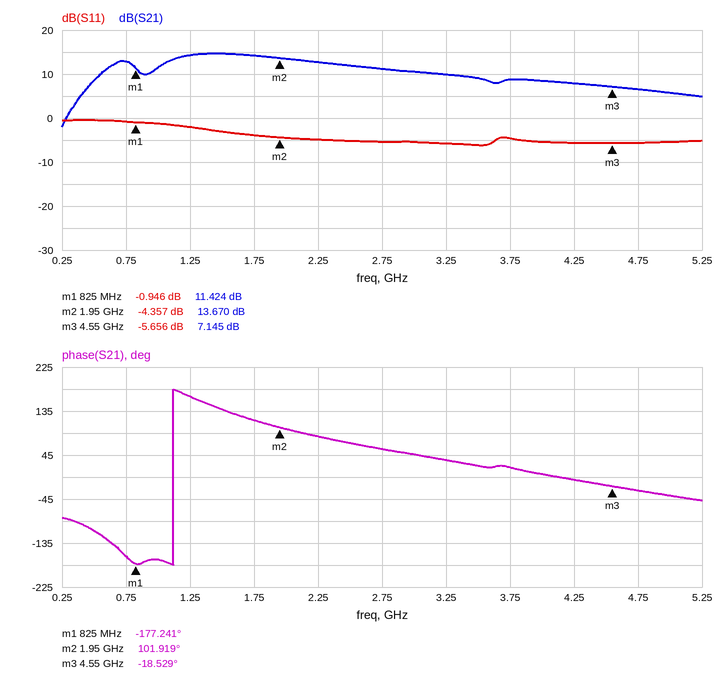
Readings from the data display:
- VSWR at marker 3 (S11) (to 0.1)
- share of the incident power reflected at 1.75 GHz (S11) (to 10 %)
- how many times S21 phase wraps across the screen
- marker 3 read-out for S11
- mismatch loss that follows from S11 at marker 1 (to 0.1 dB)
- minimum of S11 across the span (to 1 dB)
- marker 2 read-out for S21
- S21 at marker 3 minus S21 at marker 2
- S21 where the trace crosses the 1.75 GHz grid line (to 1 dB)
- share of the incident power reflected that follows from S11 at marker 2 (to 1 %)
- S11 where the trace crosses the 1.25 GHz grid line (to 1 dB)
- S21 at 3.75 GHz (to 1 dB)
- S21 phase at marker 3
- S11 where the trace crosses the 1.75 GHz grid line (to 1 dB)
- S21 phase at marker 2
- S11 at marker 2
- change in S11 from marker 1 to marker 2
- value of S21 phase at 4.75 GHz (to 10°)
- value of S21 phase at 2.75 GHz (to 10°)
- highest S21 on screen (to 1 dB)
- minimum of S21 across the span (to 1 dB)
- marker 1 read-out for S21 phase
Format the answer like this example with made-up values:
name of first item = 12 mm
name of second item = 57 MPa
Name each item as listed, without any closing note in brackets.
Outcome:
VSWR at marker 3 (S11) = 3.2
share of the incident power reflected at 1.75 GHz (S11) = 40 %
how many times S21 phase wraps across the screen = 1
marker 3 read-out for S11 = -5.656 dB
mismatch loss that follows from S11 at marker 1 = 7.1 dB
minimum of S11 across the span = -6 dB
marker 2 read-out for S21 = 13.670 dB
S21 at marker 3 minus S21 at marker 2 = -6.525 dB
S21 where the trace crosses the 1.75 GHz grid line = 14 dB
share of the incident power reflected that follows from S11 at marker 2 = 37 %
S11 where the trace crosses the 1.25 GHz grid line = -2 dB
S21 at 3.75 GHz = 9 dB
S21 phase at marker 3 = -18.529°
S11 where the trace crosses the 1.75 GHz grid line = -4 dB
S21 phase at marker 2 = 101.919°
S11 at marker 2 = -4.357 dB
change in S11 from marker 1 to marker 2 = -3.411 dB
value of S21 phase at 4.75 GHz = -30°
value of S21 phase at 2.75 GHz = 60°
highest S21 on screen = 15 dB
minimum of S21 across the span = -2 dB
marker 1 read-out for S21 phase = -177.241°
